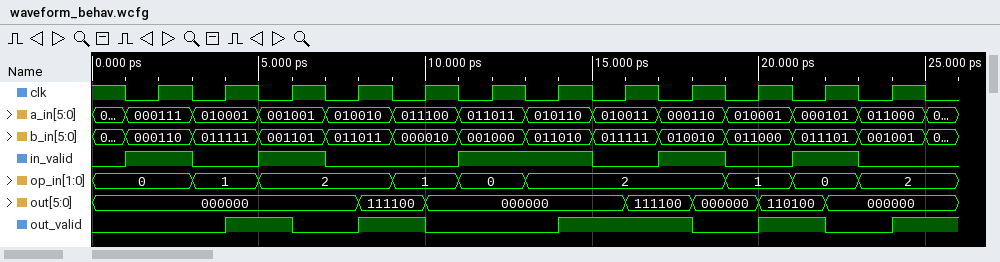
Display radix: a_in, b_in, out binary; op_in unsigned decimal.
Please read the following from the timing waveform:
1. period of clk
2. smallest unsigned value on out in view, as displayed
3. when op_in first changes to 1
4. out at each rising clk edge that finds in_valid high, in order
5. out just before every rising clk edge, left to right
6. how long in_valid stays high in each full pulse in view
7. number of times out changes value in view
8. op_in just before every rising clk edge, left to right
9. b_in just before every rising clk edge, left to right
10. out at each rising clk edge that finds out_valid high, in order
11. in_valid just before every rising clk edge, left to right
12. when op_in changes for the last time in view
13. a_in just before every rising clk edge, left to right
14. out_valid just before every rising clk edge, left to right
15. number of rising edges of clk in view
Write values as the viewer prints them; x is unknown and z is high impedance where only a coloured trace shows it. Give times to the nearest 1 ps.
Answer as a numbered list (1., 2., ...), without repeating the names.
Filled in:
1. 2 ps
2. 000000
3. 3 ps
4. 000000, 000000, 000000, 000000, 111100, 110100
5. 000000, 000000, 000000, 000000, 111100, 000000, 000000, 000000, 111100, 000000, 110100, 000000
6. 2 ps, 2 ps, 4 ps, 2 ps, 2 ps
7. 6
8. 0, 1, 2, 2, 1, 0, 2, 2, 2, 1, 0, 2
9. 000110, 011111, 001101, 011011, 000010, 001000, 011010, 011111, 010010, 011000, 011101, 001001
10. 000000, 111100, 000000, 111100, 110100
11. 1 0 1 0 0 1 1 0 1 0 1 0
12. 23 ps
13. 000111, 010001, 001001, 010010, 011100, 011011, 010110, 010011, 000110, 010001, 000101, 011000
14. 0 0 1 0 1 0 0 1 1 0 1 0
15. 12
